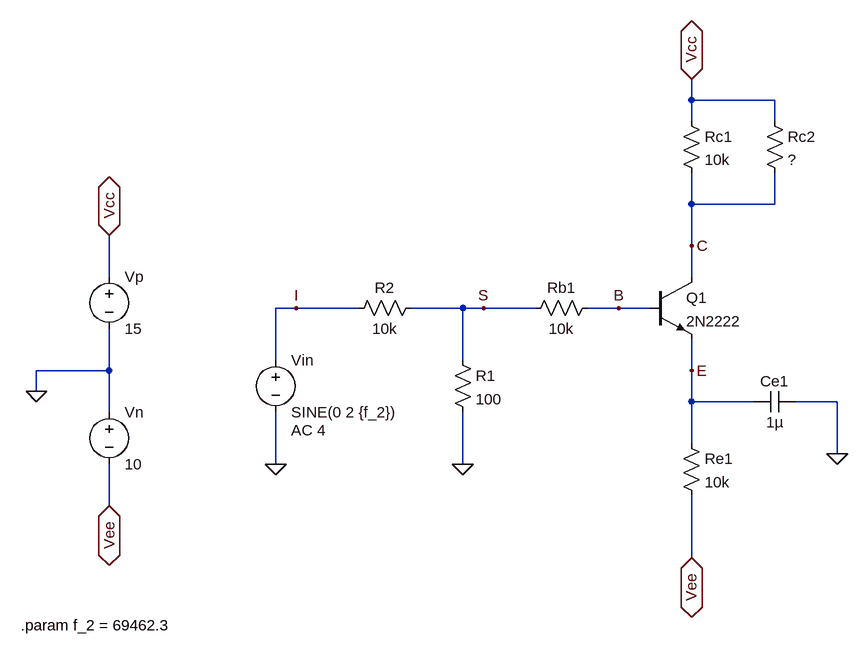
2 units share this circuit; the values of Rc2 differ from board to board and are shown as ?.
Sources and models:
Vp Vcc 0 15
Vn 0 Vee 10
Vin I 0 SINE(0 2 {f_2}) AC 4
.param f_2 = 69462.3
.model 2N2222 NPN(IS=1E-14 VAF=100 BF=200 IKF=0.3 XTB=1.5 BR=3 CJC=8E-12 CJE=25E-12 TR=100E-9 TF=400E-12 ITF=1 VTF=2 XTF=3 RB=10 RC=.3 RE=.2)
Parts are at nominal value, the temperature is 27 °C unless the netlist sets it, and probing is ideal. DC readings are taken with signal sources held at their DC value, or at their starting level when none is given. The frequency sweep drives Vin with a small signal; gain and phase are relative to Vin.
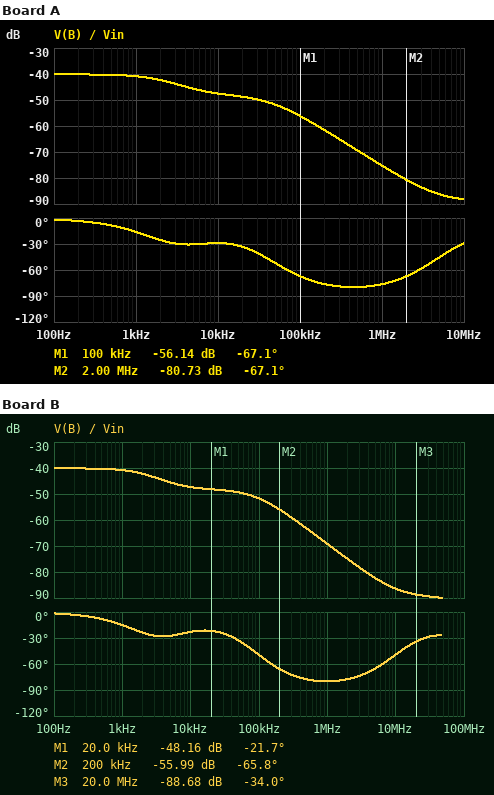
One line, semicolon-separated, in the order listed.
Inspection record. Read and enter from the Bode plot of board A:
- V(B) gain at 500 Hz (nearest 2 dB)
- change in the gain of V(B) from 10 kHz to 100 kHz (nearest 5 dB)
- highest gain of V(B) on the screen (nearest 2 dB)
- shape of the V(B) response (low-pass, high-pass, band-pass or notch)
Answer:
-40 dB; -10 dB; -40 dB; low-pass
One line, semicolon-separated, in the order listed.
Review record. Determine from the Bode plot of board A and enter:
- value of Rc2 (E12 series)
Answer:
27 kΩ
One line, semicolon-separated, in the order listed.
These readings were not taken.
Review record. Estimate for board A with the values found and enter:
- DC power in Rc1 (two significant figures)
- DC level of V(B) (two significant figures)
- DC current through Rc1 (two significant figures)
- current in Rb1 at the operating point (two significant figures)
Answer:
4.6 mW; -43 mV; 680 µA; 4.3 µA
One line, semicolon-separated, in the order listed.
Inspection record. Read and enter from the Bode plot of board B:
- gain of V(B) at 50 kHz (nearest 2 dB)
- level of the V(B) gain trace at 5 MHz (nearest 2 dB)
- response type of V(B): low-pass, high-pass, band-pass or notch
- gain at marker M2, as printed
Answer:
-50 dB; -82 dB; low-pass; -55.99 dB
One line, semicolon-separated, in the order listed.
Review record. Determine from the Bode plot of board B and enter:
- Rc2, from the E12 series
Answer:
5.6 kΩ
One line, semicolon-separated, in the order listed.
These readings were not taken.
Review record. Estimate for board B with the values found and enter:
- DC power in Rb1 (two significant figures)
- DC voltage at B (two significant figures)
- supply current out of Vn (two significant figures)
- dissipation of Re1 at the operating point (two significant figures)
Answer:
170 nW; -42 mV; 930 µA; 8.7 mW
